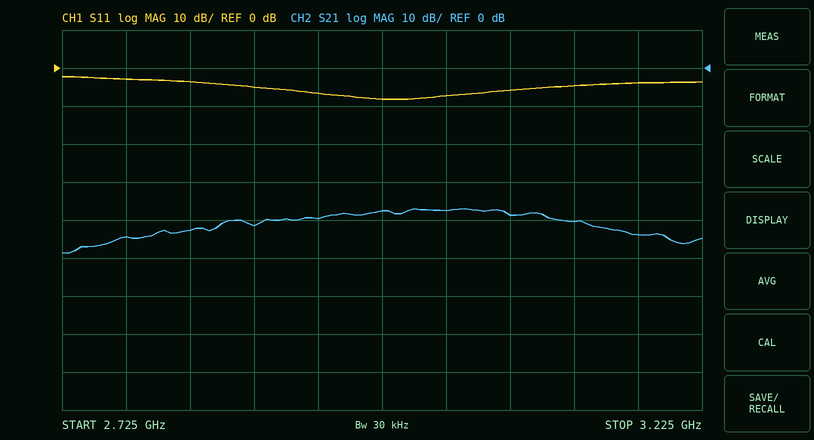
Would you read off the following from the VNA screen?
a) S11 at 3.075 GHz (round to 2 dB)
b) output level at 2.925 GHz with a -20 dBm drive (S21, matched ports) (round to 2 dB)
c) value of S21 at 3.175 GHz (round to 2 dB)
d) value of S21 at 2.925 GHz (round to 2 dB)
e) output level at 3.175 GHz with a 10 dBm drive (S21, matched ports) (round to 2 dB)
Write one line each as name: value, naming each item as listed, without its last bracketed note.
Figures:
S11 at 3.075 GHz: -6 dB
output level at 2.925 GHz with a -20 dBm drive (S21, matched ports): -60 dBm
value of S21 at 3.175 GHz: -44 dB
value of S21 at 2.925 GHz: -40 dB
output level at 3.175 GHz with a 10 dBm drive (S21, matched ports): -34 dBm
